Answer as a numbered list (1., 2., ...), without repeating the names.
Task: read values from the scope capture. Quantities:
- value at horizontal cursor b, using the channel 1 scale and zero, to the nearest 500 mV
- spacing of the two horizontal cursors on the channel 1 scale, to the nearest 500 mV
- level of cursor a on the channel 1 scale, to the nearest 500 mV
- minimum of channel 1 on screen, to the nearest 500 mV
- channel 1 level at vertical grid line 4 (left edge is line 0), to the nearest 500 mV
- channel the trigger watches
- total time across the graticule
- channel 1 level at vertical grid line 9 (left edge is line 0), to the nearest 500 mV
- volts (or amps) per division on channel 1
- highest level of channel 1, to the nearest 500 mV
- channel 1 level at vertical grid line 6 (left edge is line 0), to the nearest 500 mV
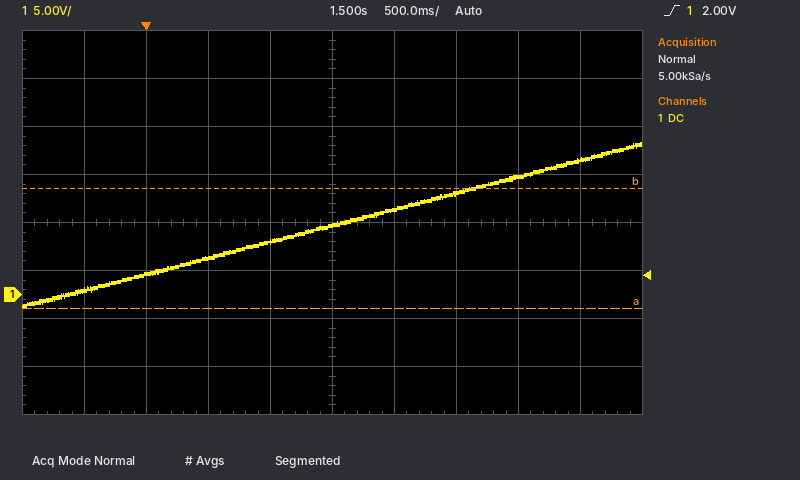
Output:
1. 11.0 V
2. 12.5 V
3. -1.5 V
4. -1.5 V
5. 5.5 V
6. channel 1
7. 5 s
8. 14.0 V
9. 5 V
10. 16.0 V
11. 9.0 V
